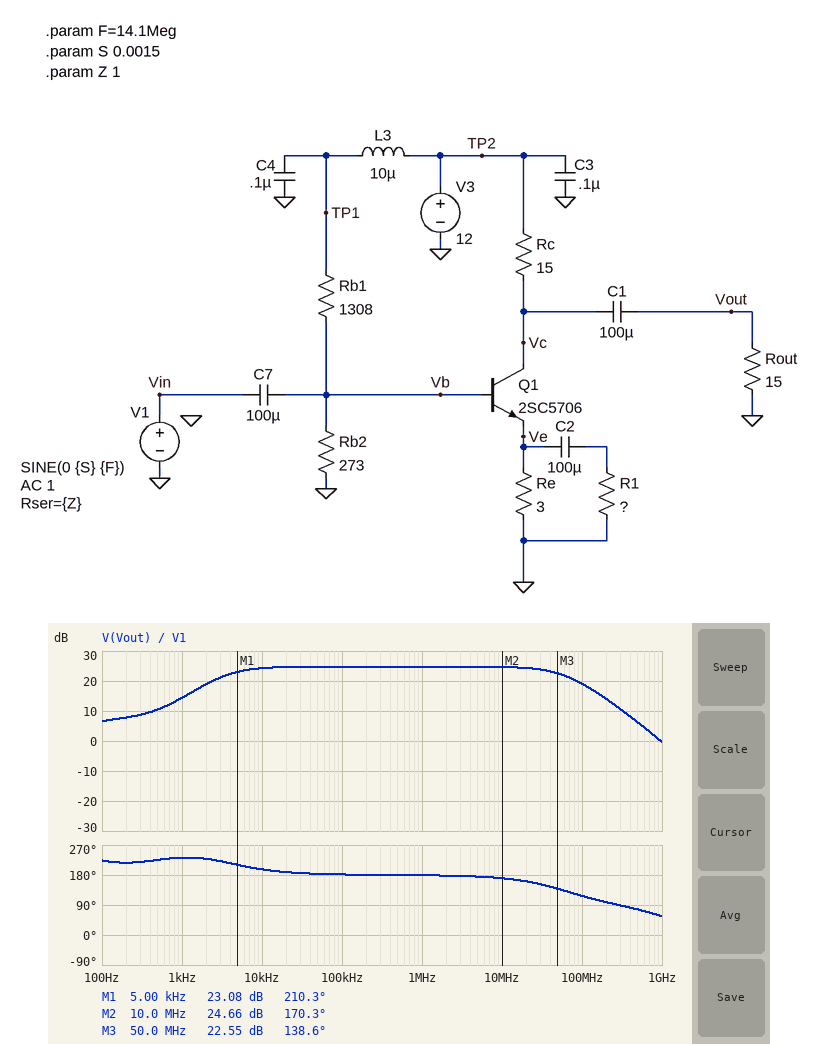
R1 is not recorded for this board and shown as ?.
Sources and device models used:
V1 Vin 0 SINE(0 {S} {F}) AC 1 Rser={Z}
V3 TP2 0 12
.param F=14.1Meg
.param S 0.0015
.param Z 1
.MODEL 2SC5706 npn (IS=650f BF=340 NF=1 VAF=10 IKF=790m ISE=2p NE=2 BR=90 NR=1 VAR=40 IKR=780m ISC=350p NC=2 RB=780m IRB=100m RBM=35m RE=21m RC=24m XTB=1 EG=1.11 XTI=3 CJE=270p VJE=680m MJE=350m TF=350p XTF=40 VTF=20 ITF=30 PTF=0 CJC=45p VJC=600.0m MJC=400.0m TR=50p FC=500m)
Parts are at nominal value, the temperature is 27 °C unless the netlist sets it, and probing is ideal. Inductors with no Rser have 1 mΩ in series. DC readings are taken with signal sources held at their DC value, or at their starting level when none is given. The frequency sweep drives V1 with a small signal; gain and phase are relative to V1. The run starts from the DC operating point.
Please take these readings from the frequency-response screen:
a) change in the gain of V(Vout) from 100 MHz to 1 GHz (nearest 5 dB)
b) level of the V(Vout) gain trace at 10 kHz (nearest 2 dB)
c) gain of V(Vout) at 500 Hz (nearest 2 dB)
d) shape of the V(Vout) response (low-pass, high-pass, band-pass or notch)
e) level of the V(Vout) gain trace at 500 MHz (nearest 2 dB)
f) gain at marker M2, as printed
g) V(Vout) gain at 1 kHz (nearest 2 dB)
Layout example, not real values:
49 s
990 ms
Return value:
-20 dB
24 dB
10 dB
band-pass
6 dB
24.66 dB
14 dB
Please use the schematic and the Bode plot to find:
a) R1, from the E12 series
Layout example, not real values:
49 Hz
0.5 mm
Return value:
0.33 Ω
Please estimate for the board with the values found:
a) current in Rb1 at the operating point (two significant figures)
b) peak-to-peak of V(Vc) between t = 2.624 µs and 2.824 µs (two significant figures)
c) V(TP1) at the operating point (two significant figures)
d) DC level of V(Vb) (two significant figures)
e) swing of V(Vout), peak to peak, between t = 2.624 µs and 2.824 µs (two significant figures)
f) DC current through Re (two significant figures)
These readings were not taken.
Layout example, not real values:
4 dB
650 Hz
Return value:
7.8 mA
51 mV
12 V
1.8 V
51 mV
380 mA
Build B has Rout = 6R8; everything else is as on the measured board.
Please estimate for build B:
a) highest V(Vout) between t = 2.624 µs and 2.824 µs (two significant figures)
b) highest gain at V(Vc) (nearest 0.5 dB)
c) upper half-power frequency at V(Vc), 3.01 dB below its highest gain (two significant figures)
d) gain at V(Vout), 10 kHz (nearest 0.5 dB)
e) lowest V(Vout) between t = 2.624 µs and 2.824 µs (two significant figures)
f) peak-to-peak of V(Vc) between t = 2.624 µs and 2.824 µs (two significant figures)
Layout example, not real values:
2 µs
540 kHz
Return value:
16 mV
21.0 dB
67 MHz
20.5 dB
-16 mV
32 mV
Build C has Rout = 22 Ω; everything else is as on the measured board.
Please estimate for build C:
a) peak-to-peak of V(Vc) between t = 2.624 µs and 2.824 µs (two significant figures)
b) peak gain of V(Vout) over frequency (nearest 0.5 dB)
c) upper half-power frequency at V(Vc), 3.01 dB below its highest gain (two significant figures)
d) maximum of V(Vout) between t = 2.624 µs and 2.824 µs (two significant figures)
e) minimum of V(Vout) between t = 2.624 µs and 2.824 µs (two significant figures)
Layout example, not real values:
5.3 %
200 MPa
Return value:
60 mV
26.0 dB
59 MHz
30 mV
-30 mV
